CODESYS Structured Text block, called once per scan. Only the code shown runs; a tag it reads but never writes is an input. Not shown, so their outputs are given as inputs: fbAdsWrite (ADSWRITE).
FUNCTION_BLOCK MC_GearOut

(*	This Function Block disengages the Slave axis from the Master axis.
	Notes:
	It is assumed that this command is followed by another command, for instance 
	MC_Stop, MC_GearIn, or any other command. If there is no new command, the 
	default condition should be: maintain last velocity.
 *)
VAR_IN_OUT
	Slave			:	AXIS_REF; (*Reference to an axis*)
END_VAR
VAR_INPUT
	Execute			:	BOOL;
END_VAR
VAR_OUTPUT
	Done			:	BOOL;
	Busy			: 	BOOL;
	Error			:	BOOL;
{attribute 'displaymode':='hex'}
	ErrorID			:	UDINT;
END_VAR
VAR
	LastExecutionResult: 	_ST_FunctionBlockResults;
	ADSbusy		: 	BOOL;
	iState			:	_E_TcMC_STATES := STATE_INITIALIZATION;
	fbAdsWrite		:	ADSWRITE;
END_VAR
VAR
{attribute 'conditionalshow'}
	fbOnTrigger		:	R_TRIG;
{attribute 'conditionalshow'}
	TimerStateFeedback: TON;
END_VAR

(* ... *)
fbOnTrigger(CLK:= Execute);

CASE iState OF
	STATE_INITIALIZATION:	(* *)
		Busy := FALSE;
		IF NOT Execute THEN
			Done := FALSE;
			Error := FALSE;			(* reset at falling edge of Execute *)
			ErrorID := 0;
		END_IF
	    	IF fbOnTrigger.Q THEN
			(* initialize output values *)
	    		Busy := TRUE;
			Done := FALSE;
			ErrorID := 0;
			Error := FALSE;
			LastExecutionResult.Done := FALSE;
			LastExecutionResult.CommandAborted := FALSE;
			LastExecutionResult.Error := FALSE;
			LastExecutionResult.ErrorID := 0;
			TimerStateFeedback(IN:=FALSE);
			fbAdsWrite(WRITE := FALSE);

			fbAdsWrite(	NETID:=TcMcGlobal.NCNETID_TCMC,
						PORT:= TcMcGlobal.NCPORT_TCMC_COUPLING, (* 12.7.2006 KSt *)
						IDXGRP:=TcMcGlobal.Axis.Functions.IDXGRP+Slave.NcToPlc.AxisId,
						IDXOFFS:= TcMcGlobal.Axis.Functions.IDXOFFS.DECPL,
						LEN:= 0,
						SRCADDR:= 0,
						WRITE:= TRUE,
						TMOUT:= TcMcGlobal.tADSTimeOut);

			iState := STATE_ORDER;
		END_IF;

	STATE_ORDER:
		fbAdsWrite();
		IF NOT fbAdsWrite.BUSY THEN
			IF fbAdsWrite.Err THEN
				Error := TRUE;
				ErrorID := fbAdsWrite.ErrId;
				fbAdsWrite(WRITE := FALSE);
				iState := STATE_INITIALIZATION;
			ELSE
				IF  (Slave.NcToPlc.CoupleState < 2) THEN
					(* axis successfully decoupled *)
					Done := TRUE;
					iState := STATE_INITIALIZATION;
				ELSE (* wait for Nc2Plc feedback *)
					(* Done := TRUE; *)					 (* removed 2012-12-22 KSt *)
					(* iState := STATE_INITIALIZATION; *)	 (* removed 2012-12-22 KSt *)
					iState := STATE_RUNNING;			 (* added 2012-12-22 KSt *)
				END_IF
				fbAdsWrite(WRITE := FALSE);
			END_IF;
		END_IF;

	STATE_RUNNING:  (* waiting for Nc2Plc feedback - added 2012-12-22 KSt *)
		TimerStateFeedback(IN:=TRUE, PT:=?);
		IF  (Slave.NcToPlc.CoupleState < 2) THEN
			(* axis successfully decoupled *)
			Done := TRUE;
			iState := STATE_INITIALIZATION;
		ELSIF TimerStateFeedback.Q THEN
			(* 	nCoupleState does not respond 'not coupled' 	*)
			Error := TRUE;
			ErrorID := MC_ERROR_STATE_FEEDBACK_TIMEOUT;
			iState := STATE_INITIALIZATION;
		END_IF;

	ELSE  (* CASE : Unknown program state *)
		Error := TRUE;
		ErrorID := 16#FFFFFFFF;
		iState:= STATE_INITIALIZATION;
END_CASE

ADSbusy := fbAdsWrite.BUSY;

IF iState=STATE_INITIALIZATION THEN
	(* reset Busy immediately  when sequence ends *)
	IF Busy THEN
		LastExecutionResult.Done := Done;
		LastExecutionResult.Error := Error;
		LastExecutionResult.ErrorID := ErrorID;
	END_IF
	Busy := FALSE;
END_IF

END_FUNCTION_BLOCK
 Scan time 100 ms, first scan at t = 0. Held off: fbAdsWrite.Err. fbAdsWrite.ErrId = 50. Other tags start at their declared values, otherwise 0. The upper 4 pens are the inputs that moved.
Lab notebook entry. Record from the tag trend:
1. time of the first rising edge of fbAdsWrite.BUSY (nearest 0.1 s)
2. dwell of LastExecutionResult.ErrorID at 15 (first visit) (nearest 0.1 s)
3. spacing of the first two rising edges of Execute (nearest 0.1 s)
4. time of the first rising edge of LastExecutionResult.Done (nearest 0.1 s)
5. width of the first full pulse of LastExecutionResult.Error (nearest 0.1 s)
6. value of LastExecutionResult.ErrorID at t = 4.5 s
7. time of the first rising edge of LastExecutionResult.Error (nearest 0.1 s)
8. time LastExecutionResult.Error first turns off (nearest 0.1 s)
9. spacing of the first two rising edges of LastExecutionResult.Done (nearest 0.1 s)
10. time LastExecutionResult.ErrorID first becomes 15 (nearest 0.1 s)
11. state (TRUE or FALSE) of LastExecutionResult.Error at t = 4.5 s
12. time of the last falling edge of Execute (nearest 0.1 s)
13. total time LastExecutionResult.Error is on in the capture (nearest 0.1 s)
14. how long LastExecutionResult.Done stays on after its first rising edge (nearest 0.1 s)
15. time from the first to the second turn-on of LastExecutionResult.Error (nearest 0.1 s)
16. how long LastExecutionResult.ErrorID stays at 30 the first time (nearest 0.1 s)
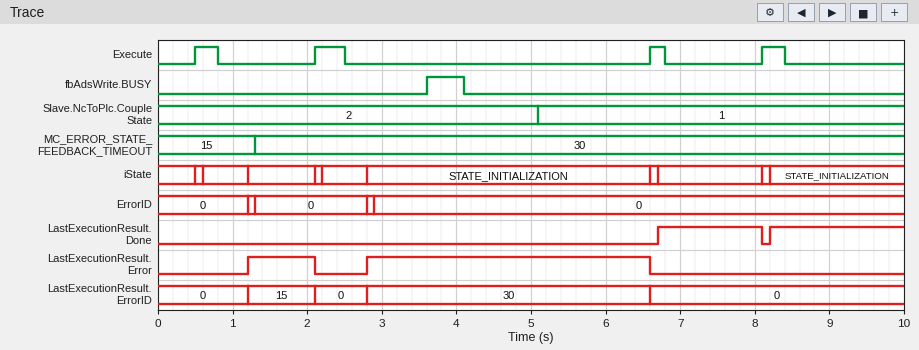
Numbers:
3.6 s
0.9 s
1.6 s
6.7 s
0.9 s
30
1.2 s
2.1 s
1.5 s
1.2 s
TRUE
8.4 s
4.7 s
1.4 s
1.6 s
3.8 s
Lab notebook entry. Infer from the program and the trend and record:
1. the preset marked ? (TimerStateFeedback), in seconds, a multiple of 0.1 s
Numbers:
0.5 s
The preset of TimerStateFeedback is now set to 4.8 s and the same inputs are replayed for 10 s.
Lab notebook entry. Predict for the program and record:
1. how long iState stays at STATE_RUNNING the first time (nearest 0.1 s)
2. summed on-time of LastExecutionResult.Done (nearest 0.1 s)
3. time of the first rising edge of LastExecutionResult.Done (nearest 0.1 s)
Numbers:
4.5 s
4.7 s
5.1 s
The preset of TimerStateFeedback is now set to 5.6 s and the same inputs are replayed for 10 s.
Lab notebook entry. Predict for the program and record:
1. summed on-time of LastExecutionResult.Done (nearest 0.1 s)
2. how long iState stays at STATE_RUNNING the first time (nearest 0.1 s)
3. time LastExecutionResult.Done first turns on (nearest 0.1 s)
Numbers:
4.7 s
4.5 s
5.1 s
